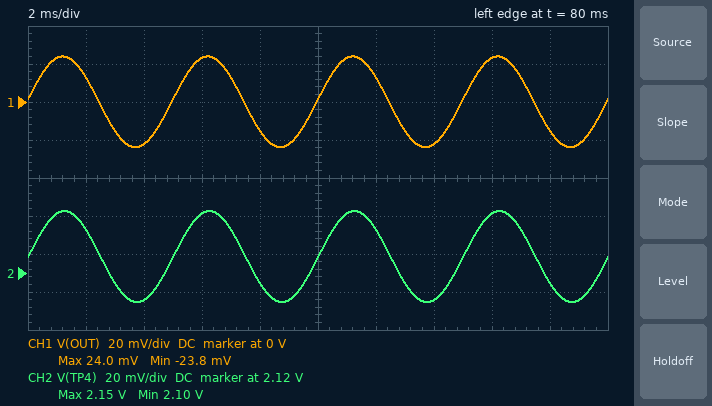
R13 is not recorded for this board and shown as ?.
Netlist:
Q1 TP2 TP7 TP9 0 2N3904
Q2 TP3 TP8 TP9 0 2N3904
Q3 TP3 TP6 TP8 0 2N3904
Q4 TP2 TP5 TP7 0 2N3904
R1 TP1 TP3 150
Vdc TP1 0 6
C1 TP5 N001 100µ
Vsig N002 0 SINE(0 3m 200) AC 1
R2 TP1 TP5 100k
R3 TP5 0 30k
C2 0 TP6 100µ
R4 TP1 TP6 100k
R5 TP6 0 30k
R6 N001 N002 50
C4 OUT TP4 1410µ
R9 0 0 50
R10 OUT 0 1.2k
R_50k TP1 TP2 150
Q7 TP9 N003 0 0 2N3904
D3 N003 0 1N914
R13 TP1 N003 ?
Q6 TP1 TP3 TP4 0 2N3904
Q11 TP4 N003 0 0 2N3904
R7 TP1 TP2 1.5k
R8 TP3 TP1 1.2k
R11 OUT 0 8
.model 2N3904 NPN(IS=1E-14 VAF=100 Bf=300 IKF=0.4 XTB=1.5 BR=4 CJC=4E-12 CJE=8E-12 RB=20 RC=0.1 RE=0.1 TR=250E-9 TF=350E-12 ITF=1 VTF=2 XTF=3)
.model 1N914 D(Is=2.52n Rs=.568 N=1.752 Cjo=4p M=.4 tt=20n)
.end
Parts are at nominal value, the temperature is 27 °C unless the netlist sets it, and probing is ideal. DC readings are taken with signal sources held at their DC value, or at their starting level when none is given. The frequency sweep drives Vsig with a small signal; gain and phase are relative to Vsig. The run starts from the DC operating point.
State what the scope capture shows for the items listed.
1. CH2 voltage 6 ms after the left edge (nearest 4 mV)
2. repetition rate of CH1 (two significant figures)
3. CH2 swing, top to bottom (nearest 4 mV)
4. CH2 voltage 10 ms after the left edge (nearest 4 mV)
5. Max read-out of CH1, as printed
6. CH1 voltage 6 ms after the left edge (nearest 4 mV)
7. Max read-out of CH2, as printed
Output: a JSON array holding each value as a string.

["2.152 V", "200 Hz", "48 mV", "2.128 V", "24.0 mV", "24 mV", "2.15 V"]
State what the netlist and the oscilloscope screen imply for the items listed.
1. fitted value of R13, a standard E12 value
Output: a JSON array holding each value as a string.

["56 Ω"]
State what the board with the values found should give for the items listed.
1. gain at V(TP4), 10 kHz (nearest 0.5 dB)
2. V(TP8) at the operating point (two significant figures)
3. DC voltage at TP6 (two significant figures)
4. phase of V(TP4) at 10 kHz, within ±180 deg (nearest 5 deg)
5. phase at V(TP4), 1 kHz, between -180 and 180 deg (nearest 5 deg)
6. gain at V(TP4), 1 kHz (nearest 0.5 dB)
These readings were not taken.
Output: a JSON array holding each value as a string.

["18.0 dB", "790 mV", "1.4 V", "0 deg", "0 deg", "18.0 dB"]
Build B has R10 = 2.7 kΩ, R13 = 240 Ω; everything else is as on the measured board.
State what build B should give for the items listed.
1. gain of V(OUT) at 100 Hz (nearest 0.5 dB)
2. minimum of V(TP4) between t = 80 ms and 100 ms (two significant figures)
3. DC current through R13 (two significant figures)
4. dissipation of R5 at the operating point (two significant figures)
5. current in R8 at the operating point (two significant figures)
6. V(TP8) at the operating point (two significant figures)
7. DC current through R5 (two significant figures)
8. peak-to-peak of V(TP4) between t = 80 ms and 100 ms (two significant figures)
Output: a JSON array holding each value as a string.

["17.0 dB", "4.1 V", "22 mA", "64 µW", "990 µA", "820 mV", "46 µA", "43 mV"]
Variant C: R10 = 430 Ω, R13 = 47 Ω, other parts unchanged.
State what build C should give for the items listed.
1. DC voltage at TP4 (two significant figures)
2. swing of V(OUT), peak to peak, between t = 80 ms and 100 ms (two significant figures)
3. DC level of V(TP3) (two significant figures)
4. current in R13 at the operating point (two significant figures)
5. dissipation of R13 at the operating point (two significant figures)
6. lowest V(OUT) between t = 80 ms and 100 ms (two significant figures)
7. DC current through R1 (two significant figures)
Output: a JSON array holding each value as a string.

["2.0 V", "47 mV", "2.8 V", "110 mA", "560 mW", "-23 mV", "21 mA"]
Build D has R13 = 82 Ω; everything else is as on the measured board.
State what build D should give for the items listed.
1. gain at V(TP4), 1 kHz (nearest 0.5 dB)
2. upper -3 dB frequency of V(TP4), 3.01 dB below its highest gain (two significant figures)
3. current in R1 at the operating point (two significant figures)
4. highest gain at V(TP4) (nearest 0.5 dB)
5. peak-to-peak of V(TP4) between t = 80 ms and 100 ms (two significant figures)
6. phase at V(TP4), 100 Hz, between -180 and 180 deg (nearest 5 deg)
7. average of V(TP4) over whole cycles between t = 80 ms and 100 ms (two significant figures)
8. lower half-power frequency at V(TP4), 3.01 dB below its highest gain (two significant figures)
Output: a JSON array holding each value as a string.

["18.5 dB", "400 kHz", "18 mA", "19.5 dB", "49 mV", "0 deg", "2.5 V", "78 mHz"]
